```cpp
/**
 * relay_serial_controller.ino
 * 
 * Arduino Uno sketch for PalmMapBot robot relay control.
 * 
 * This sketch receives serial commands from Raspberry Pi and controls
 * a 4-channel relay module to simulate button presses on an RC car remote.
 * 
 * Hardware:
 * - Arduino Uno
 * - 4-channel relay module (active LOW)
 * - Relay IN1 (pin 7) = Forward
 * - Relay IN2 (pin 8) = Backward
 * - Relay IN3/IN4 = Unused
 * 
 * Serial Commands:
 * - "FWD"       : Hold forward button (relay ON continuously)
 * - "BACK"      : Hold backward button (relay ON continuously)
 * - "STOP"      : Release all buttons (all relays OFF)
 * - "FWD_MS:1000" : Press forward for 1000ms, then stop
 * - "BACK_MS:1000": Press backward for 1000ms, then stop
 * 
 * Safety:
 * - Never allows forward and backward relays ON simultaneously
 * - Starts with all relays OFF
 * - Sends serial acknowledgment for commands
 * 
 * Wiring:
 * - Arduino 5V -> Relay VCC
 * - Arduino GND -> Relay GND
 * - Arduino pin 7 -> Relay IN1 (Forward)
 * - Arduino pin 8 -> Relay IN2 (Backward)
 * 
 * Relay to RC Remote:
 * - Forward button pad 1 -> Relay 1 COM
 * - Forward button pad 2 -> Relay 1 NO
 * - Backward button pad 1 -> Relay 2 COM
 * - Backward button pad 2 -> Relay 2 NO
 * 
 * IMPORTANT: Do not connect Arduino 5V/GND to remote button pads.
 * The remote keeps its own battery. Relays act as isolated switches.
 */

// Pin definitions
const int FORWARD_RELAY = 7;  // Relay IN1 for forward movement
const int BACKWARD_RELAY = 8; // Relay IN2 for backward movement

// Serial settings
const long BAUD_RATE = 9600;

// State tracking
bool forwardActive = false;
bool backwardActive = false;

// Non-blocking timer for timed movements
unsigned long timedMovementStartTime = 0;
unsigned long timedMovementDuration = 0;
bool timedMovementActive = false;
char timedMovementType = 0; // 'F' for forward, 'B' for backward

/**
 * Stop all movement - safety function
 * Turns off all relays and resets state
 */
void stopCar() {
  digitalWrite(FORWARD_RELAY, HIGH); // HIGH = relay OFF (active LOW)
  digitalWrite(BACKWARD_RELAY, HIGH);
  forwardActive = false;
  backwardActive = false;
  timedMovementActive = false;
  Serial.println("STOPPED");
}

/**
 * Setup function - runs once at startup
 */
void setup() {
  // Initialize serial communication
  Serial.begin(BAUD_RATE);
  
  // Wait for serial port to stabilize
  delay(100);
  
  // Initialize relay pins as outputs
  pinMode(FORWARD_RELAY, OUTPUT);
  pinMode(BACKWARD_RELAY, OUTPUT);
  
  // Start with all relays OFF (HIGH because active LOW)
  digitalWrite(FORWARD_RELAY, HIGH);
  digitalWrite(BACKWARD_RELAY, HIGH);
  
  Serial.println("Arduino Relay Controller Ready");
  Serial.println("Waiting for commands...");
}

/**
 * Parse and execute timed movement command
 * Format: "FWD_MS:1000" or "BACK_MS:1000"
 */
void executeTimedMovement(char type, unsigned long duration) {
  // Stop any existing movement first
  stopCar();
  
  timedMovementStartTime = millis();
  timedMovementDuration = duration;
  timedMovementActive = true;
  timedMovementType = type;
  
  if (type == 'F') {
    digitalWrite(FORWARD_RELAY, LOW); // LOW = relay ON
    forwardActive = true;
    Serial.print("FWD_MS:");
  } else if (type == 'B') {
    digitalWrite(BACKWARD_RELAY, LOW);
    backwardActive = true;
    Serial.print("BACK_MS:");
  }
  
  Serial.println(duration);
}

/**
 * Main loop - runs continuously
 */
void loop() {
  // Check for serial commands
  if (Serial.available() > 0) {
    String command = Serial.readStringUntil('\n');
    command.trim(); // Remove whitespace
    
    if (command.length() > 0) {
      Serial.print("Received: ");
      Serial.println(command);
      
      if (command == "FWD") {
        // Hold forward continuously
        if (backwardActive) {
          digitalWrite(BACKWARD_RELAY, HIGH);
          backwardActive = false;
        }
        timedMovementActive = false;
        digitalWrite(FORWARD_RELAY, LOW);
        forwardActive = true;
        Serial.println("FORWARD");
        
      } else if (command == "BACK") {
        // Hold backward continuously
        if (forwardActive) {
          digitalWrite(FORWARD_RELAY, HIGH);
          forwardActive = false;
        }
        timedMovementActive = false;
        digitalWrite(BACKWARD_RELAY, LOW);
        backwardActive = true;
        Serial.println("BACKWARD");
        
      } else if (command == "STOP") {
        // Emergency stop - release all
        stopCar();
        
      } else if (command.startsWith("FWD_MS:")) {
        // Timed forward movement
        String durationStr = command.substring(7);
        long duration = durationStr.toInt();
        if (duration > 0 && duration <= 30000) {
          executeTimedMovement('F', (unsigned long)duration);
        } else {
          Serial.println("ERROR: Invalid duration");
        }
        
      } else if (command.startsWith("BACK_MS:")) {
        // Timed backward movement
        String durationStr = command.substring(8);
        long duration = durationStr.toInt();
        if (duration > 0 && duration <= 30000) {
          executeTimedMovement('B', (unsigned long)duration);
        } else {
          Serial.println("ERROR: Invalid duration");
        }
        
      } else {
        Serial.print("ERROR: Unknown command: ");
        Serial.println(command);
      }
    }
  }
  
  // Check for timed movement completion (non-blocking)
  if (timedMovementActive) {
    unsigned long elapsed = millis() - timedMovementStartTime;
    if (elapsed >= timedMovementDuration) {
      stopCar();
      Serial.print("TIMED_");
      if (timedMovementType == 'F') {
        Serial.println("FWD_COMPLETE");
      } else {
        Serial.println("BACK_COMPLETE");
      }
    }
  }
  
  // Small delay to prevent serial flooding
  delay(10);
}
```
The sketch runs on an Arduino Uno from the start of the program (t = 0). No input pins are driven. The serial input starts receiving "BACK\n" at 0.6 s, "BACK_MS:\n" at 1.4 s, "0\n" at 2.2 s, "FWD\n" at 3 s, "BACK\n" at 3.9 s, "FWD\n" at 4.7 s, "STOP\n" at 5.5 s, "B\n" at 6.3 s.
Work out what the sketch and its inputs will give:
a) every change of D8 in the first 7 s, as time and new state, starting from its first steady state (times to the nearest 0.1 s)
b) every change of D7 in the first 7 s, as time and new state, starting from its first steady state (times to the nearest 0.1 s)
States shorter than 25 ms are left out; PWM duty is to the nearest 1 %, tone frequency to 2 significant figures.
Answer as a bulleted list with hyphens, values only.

- 0.1 s high; 0.6 s low; 3 s high; 3.9 s low; 4.7 s high
- 0.1 s high; 3 s low; 3.9 s high; 4.7 s low; 5.5 s high
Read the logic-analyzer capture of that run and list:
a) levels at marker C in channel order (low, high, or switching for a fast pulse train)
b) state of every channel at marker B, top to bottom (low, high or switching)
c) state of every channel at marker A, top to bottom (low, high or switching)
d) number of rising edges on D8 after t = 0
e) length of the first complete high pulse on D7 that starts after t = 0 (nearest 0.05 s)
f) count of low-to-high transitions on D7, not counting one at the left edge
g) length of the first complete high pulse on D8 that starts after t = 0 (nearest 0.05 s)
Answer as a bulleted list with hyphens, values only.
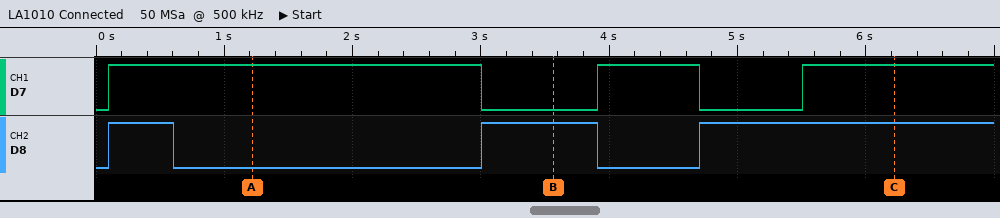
- D7 high, D8 high
- D7 low, D8 high
- D7 high, D8 low
- 3
- 2.90 s
- 3
- 0.50 s
